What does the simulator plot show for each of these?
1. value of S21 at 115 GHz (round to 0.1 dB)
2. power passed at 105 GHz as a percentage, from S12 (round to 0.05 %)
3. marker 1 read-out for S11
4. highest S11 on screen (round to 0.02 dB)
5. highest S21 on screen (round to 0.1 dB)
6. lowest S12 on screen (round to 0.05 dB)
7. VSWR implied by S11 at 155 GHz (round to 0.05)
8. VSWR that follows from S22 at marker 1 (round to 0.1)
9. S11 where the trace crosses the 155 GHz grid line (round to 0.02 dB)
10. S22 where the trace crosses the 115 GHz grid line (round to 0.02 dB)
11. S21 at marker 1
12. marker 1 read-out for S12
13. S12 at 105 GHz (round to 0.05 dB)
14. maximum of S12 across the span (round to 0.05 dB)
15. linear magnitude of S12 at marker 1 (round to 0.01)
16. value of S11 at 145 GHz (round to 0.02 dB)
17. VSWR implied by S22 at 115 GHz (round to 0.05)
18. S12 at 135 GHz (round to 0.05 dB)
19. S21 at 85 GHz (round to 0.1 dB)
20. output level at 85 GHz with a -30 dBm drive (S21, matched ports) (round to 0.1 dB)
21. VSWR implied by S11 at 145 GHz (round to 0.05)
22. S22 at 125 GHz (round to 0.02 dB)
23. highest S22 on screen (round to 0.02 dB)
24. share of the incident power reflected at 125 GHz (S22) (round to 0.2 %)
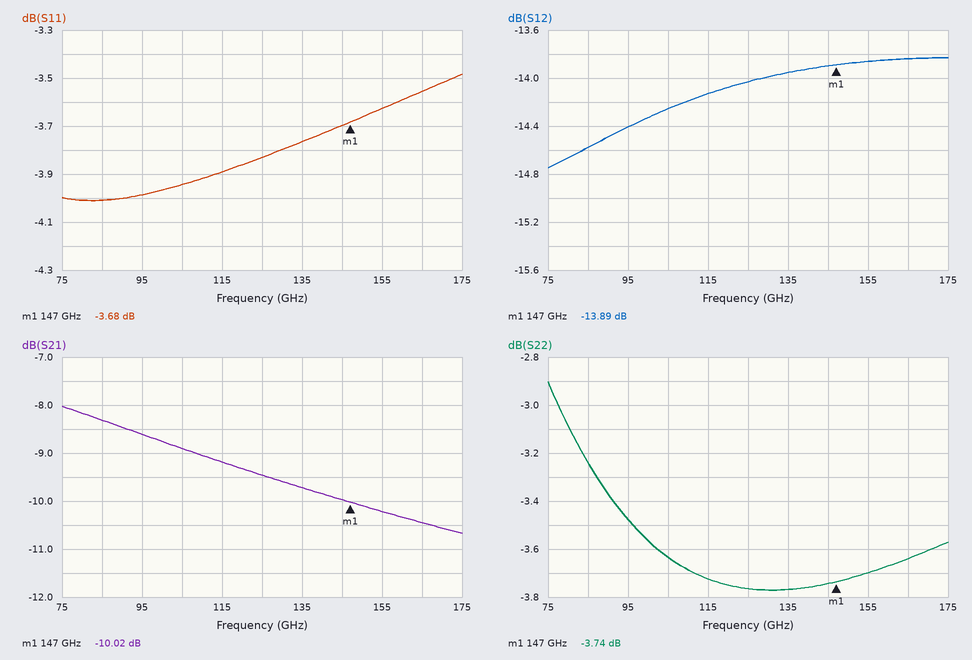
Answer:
-9.2 dB
3.75 %
-3.68 dB
-3.48 dB
-8.0 dB
-14.75 dB
4.85
4.7
-3.62 dB
-3.72 dB
-10.02 dB
-13.89 dB
-14.25 dB
-13.85 dB
0.20
-3.70 dB
4.75
-13.95 dB
-8.3 dB
-38.3 dBm
4.75
-3.76 dB
-2.90 dB
42.0 %
